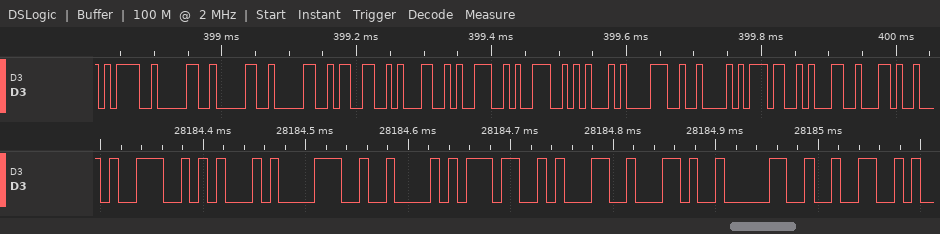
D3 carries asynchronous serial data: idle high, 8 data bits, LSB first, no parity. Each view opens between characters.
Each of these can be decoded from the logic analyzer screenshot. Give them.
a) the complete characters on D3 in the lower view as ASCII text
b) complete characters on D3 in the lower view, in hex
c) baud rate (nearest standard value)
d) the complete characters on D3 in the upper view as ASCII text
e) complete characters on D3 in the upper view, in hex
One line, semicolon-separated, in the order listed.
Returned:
"9E8B71,02"; 39, 45, 38, 42, 37, 31, 2C, 30, 32; 115200 baud; "=0003199E8B71,"; 3D, 30, 30, 30, 33, 31, 39, 39, 45, 38, 42, 37, 31, 2C
